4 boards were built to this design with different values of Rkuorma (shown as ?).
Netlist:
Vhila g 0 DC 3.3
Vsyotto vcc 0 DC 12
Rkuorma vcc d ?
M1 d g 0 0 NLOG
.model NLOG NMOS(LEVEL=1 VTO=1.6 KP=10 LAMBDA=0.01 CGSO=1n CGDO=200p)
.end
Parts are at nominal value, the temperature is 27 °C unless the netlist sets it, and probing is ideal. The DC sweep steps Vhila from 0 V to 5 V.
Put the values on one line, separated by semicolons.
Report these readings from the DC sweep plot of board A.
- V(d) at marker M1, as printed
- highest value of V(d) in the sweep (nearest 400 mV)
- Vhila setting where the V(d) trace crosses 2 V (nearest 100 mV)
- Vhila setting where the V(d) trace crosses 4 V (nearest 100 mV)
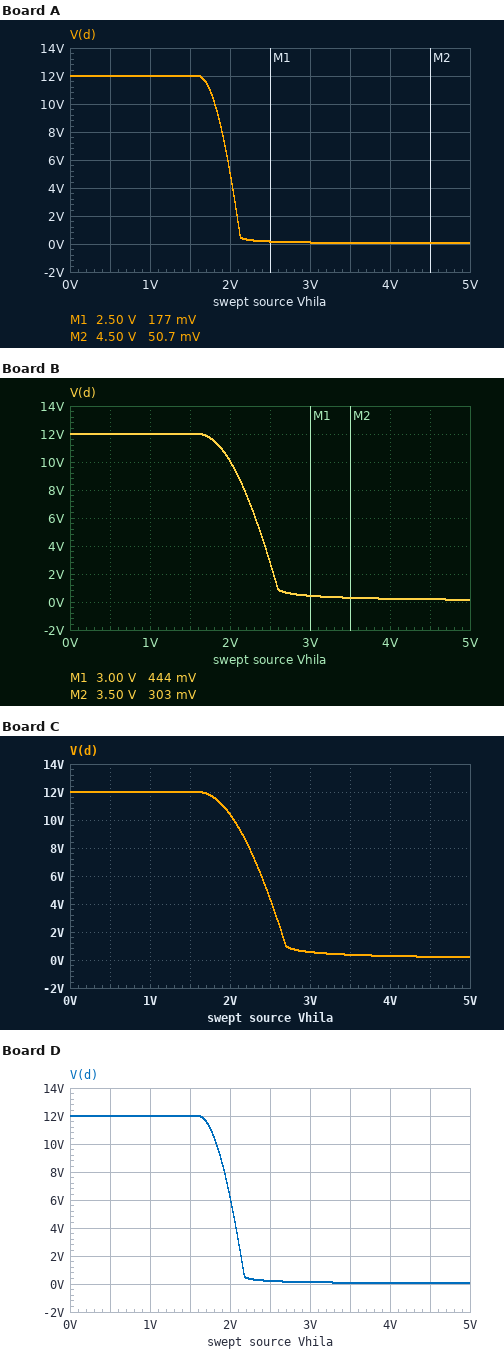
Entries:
177 mV; 12.0 V; 2.1 V; 2.0 V
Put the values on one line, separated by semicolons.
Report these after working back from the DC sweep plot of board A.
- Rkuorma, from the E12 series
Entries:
8.2 Ω
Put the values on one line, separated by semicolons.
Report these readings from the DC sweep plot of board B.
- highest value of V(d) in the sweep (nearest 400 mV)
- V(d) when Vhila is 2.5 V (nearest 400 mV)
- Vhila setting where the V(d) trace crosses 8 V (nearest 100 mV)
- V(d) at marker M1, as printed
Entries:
12.0 V; 2.8 V; 2.2 V; 444 mV
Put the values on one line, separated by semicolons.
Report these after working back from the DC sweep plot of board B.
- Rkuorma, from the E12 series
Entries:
2.2 Ω
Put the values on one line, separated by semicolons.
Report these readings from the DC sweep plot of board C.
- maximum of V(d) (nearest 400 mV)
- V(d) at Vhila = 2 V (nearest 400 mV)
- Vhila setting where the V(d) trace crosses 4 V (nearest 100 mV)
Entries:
12.0 V; 10.4 V; 2.5 V
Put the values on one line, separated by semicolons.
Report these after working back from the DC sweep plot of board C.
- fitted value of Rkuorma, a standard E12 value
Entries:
1.8 Ω
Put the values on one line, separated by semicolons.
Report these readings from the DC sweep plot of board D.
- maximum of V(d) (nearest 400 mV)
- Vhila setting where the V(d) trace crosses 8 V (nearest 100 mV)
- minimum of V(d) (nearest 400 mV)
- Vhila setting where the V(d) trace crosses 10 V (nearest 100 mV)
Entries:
12.0 V; 1.9 V; 0 V; 1.8 V
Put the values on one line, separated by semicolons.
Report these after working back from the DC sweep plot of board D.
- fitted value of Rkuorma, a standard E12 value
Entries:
6.8 Ω
